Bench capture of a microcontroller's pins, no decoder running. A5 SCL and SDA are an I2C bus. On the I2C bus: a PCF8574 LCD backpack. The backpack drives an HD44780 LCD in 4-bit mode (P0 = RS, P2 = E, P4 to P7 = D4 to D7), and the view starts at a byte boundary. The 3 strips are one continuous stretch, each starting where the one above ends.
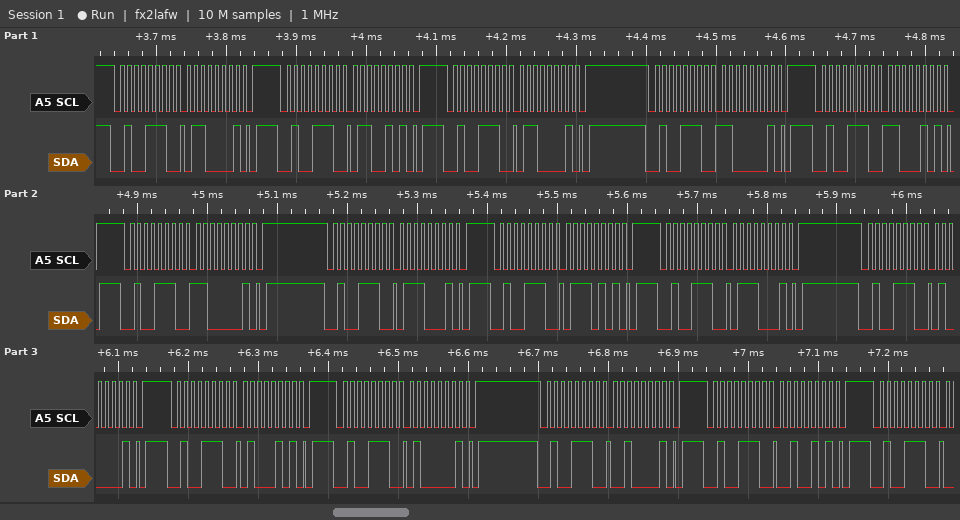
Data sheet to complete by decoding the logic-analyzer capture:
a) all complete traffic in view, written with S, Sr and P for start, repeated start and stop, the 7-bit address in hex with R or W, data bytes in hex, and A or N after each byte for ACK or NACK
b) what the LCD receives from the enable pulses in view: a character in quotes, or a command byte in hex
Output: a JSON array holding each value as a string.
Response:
["S 27W A 61 A P S 27W A 65 A P S 27W A 61 A P S 27W A C1 A P S 27W A C5 A P S 27W A C1 A P S 27W A 71 A P S 27W A 75 A P S 27W A 71 A P S 27W A 41 A P S 27W A 45 A P S 27W A 41 A P S 27W A 21 A P S 27W A 25 A P S 27W A", "'l' 't'"]
